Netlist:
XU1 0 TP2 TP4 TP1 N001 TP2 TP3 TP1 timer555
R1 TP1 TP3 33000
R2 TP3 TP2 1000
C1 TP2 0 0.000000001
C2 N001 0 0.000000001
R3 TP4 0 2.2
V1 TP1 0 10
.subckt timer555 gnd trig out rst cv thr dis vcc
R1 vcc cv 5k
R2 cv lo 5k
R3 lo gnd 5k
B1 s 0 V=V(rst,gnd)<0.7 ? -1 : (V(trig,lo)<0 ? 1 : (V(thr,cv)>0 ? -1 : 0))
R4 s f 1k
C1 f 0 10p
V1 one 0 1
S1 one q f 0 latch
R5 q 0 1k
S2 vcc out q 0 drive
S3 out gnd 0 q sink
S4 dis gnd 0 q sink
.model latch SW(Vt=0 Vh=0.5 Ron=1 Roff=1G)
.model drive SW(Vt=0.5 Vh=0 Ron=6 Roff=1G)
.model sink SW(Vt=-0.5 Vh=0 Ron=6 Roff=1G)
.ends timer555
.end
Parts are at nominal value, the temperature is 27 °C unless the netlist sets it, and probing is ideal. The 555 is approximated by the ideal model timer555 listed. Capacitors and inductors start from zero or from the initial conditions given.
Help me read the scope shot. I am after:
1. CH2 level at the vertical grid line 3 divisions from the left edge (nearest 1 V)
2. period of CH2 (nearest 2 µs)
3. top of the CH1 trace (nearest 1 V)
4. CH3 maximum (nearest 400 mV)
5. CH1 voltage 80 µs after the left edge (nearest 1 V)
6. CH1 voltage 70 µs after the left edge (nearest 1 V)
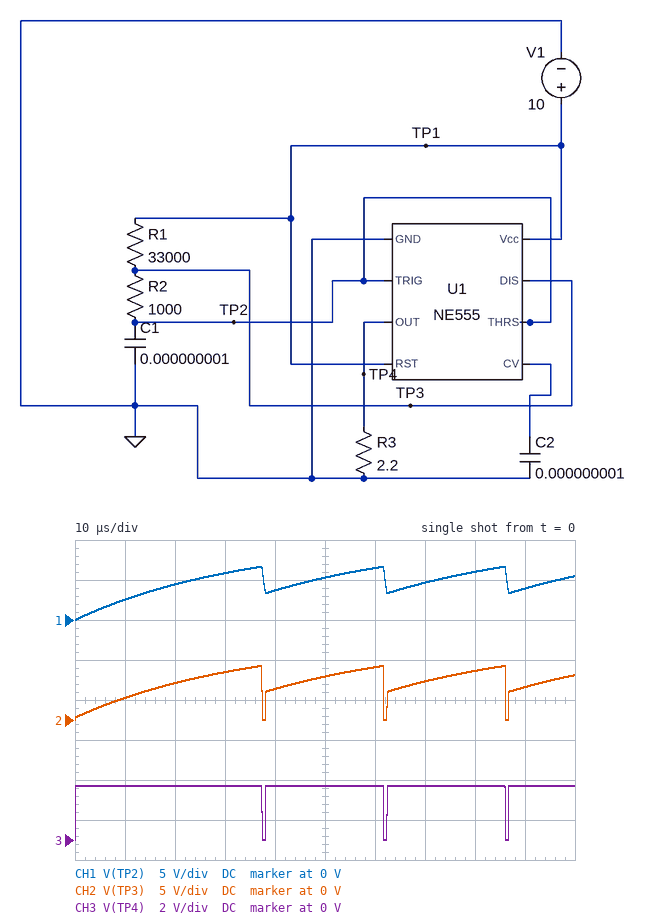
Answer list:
6 V
24 µs
7 V
2.8 V
6 V
5 V
